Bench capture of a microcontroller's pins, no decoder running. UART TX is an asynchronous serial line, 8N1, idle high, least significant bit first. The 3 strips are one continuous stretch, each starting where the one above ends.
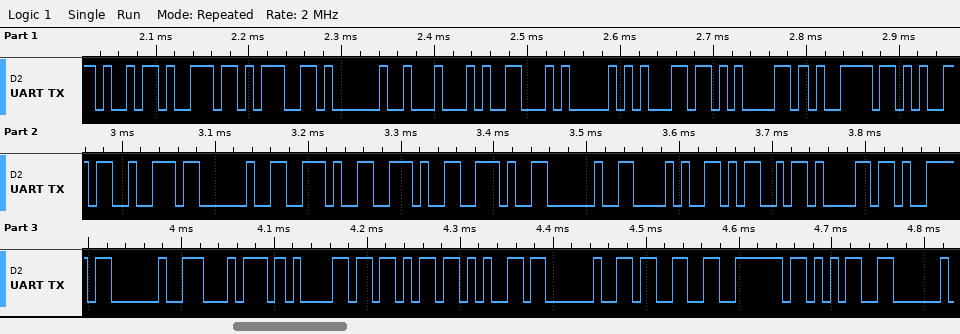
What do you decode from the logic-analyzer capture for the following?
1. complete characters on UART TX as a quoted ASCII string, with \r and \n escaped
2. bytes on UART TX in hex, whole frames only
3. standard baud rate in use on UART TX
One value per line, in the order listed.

"ing DFPlayer ... (May take 3~5"
0x69 0x6E 0x67 0x20 0x44 0x46 0x50 0x6C 0x61 0x79 0x65 0x72 0x20 0x2E 0x2E 0x2E 0x20 0x28 0x4D 0x61 0x79 0x20 0x74 0x61 0x6B 0x65 0x20 0x33 0x7E 0x35
115200 baud
